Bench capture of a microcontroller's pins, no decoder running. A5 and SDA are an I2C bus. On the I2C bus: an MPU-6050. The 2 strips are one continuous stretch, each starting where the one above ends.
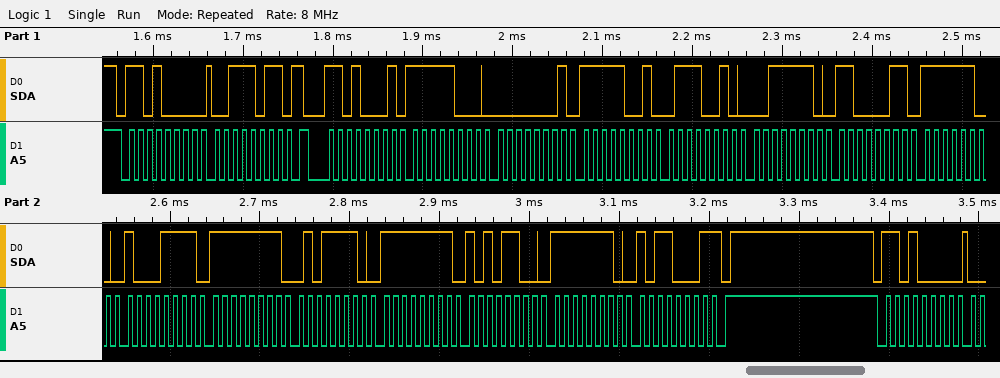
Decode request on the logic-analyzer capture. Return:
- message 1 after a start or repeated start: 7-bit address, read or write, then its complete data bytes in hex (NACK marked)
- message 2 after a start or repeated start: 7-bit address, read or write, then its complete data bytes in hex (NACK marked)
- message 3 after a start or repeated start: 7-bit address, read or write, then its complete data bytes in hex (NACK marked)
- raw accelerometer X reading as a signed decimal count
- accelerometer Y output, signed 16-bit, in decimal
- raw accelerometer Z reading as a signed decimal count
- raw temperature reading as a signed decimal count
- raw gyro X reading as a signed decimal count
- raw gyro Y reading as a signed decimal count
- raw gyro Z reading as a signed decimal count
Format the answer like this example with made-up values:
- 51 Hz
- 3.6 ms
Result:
- 0x68 write: 3B
- 0x68 read: F8 01 F9 72 3E C3 FC 8F FF 5E FF AC FE B1 NACK
- 0x68 write
- -2047
- -1678
- 16067
- -881
- -162
- -84
- -335
